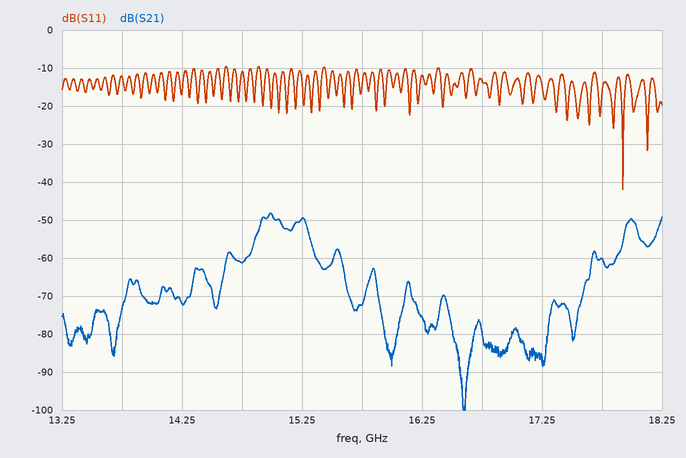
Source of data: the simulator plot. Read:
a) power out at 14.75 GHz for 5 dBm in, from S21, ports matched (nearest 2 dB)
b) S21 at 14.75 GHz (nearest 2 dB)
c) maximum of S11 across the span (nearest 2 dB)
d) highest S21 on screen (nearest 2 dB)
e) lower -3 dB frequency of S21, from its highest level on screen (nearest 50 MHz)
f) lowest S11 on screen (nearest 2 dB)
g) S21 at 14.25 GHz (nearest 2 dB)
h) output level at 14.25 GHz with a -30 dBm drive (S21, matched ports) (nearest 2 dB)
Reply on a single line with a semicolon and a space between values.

-56 dBm; -62 dB; -10 dB; -48 dB; 14.90 GHz; -42 dB; -72 dB; -102 dBm
